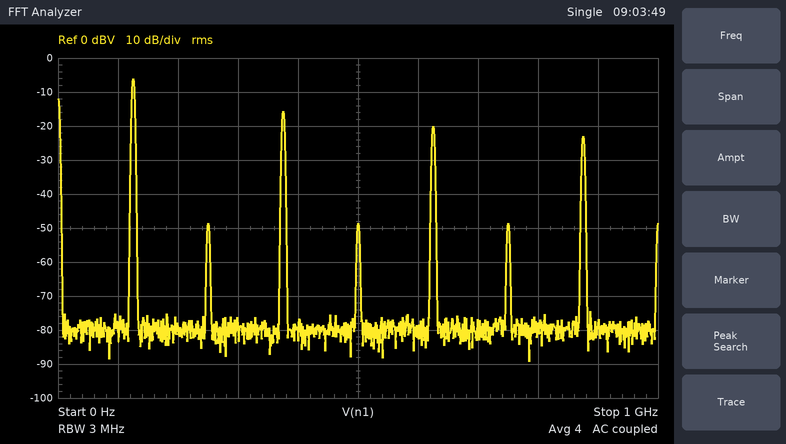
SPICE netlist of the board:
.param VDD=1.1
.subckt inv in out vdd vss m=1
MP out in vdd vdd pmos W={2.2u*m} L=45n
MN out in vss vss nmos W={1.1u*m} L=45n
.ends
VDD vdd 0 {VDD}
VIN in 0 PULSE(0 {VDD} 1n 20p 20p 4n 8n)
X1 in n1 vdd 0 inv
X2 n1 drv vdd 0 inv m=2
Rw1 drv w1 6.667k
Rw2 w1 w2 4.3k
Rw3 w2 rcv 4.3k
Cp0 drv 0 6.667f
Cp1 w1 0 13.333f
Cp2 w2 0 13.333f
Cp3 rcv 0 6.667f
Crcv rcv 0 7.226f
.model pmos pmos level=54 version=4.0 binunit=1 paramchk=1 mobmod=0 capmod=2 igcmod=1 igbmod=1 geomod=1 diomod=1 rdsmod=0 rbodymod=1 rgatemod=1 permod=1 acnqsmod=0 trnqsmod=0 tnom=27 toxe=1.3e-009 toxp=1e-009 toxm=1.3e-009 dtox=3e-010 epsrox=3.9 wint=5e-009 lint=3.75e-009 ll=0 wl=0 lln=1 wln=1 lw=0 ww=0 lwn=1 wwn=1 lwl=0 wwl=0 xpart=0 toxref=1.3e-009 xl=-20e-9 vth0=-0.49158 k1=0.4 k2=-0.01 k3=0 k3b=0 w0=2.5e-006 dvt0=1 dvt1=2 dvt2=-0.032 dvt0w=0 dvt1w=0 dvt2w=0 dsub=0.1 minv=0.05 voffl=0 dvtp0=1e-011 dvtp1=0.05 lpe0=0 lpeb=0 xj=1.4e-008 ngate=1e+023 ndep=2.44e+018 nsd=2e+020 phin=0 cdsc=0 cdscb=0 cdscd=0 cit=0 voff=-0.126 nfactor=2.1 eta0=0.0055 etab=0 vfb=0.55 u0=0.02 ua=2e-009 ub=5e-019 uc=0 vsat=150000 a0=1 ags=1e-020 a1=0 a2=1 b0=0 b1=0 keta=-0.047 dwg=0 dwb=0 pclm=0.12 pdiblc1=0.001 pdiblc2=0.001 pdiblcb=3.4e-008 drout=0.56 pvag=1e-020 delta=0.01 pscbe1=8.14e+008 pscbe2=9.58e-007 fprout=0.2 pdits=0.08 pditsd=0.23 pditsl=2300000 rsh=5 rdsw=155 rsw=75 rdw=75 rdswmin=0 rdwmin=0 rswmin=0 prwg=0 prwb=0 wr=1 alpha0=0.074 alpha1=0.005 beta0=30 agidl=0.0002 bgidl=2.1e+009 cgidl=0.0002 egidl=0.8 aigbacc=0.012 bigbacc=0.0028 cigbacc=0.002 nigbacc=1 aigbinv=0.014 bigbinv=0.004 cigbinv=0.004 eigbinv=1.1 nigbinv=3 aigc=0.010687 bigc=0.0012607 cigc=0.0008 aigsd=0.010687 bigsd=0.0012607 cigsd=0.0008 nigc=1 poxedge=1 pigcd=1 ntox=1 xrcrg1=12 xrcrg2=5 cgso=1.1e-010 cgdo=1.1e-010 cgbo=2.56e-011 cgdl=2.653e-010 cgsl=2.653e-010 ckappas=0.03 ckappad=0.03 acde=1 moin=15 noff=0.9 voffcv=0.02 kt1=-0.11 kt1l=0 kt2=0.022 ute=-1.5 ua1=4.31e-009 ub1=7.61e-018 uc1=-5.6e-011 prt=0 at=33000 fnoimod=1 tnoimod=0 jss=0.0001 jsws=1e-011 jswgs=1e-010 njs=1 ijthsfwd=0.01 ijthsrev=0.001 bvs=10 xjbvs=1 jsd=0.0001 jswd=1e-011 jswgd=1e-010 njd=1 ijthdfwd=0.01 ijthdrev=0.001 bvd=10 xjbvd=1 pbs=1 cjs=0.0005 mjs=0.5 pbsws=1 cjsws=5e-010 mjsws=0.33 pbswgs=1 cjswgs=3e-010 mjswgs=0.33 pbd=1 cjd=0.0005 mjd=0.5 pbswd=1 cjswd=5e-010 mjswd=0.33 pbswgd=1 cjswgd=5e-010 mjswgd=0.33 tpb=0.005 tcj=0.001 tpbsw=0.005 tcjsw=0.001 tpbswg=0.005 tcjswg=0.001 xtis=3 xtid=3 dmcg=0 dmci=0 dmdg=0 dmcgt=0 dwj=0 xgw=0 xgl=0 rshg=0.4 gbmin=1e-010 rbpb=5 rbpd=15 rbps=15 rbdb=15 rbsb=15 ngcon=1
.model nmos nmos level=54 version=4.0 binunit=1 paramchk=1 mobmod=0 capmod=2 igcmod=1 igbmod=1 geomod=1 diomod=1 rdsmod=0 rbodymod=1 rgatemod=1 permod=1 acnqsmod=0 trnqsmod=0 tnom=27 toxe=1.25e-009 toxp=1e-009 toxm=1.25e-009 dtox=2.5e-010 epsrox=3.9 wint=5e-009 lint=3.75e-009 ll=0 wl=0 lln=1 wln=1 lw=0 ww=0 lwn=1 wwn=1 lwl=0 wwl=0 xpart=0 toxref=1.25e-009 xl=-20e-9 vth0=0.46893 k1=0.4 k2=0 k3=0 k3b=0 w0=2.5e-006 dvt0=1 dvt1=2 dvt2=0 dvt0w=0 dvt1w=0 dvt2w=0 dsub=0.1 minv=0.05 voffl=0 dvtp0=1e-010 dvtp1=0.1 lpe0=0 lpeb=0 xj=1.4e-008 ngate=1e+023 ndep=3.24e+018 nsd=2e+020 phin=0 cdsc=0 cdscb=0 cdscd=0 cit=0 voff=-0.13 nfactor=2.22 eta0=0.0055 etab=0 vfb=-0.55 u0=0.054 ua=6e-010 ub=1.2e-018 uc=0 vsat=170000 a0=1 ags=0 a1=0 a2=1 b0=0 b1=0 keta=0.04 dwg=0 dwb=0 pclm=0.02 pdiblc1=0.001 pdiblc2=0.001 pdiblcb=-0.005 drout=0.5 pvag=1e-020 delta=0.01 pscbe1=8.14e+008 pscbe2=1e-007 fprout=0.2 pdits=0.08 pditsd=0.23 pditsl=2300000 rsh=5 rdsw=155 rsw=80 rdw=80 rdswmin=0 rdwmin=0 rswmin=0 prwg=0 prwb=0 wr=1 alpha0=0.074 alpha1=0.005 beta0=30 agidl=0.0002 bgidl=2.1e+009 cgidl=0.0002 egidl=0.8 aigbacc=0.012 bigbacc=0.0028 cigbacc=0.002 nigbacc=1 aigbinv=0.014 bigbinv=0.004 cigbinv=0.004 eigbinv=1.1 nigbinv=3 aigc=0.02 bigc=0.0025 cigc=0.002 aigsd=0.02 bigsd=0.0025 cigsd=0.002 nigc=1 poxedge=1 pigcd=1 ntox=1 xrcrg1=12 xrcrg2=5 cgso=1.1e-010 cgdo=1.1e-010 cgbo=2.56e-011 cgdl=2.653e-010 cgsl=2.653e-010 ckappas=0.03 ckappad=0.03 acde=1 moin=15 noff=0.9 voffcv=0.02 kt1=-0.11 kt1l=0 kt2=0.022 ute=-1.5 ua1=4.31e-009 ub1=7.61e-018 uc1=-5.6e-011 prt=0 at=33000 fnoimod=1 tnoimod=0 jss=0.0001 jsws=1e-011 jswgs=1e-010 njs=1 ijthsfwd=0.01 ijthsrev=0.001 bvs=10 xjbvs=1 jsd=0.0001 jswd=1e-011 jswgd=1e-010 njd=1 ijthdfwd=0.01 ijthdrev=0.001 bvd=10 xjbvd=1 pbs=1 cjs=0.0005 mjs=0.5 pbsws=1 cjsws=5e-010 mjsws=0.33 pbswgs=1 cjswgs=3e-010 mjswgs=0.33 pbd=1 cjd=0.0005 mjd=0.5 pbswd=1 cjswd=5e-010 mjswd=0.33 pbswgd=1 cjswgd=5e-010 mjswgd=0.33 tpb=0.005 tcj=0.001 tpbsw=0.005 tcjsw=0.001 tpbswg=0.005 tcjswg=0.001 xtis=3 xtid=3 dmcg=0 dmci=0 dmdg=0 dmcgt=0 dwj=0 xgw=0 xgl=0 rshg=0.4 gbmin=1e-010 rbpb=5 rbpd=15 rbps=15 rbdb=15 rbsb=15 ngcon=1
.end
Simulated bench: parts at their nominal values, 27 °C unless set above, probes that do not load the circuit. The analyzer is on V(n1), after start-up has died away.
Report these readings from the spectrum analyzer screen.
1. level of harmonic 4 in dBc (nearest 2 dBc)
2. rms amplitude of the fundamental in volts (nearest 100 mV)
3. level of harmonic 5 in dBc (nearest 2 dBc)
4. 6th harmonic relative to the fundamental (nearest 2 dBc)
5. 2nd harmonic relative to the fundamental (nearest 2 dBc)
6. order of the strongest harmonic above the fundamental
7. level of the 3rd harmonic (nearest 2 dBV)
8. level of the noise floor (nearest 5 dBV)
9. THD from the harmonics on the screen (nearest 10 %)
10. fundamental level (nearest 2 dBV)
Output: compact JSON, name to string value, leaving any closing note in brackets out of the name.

{"level of harmonic 4 in dBc": "-42 dBc", "rms amplitude of the fundamental in volts": "500 mV", "level of harmonic 5 in dBc": "-14 dBc", "6th harmonic relative to the fundamental": "-42 dBc", "2nd harmonic relative to the fundamental": "-42 dBc", "order of the strongest harmonic above the fundamental": "3", "level of the 3rd harmonic": "-16 dBV", "level of the noise floor": "-80 dBV", "THD from the harmonics on the screen": "40 %", "fundamental level": "-6 dBV"}
